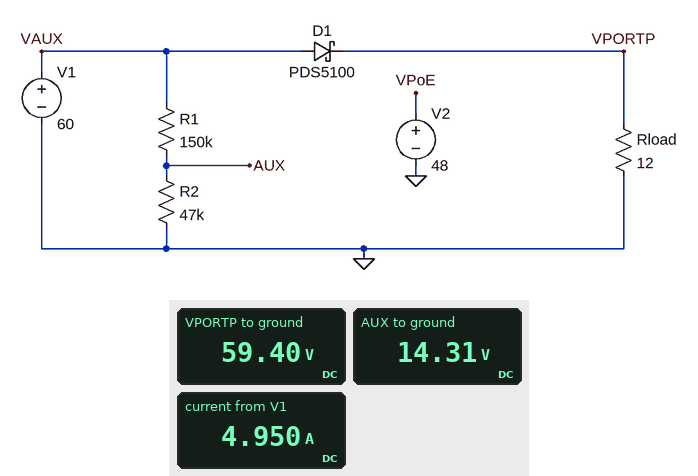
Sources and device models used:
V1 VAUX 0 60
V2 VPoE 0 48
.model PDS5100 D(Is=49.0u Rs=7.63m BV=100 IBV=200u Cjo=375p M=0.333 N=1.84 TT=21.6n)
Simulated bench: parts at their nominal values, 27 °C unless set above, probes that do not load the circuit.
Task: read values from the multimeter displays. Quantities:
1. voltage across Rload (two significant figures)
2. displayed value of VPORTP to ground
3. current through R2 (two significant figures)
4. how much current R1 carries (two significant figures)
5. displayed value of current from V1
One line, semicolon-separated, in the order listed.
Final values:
59 V; 59.40 V; 300 µA; 300 µA; 4.950 A
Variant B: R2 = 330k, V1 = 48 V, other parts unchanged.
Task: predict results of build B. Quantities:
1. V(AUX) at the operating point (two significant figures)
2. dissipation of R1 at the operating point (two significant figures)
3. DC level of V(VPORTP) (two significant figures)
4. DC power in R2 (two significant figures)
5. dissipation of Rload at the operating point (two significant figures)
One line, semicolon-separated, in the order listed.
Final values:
33 V; 1.5 mW; 47 V; 3.3 mW; 190 W
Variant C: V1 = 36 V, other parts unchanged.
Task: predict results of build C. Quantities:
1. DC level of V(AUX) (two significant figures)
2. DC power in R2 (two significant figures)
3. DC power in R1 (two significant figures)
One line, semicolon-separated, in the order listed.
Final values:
8.6 V; 1.6 mW; 5.0 mW
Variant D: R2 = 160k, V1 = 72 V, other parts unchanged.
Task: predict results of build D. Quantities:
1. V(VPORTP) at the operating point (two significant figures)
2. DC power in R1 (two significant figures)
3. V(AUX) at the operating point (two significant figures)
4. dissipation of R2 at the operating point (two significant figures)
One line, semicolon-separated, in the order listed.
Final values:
71 V; 8.1 mW; 37 V; 8.6 mW
